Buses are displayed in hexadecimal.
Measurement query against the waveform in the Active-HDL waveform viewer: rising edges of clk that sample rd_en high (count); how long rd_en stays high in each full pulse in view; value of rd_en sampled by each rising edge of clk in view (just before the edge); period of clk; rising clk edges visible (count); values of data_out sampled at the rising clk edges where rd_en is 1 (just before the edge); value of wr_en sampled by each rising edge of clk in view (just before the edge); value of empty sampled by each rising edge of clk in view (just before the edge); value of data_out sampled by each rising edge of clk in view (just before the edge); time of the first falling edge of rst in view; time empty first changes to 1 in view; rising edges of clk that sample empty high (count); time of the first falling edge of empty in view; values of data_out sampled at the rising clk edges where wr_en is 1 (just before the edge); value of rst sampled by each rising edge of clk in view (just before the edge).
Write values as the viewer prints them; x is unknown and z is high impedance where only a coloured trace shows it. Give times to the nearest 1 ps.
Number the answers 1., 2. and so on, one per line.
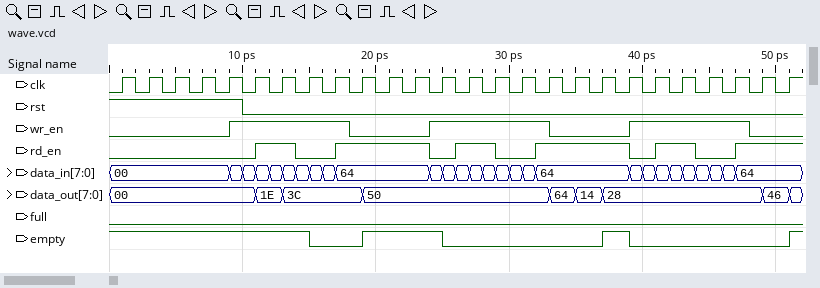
1. 13
2. 3 ps, 7 ps, 3 ps, 7 ps, 3 ps
3. 0 0 0 0 0 0 1 0 0 1 1 1 0 1 1 0 1 1 1 1 0 1 0 0 1 1
4. 2 ps
5. 26
6. 1E, 3C, 50, 50, 50, 50, 50, 64, 14, 28, 28, 28, 46
7. 0 0 0 0 0 1 1 1 1 0 0 0 1 1 1 1 1 0 0 0 1 1 1 1 0 0
8. 1 1 1 1 1 1 1 1 0 0 1 1 1 0 0 0 0 0 0 1 0 0 0 0 0 0
9. 00, 00, 00, 00, 00, 00, 1E, 3C, 3C, 3C, 50, 50, 50, 50, 50, 50, 50, 64, 14, 28, 28, 28, 28, 28, 28, 46
10. 10 ps
11. 19 ps
12. 12
13. 15 ps
14. 00, 1E, 3C, 3C, 50, 50, 50, 50, 50, 28, 28, 28, 28
15. 1 1 1 1 1 0 0 0 0 0 0 0 0 0 0 0 0 0 0 0 0 0 0 0 0 0
